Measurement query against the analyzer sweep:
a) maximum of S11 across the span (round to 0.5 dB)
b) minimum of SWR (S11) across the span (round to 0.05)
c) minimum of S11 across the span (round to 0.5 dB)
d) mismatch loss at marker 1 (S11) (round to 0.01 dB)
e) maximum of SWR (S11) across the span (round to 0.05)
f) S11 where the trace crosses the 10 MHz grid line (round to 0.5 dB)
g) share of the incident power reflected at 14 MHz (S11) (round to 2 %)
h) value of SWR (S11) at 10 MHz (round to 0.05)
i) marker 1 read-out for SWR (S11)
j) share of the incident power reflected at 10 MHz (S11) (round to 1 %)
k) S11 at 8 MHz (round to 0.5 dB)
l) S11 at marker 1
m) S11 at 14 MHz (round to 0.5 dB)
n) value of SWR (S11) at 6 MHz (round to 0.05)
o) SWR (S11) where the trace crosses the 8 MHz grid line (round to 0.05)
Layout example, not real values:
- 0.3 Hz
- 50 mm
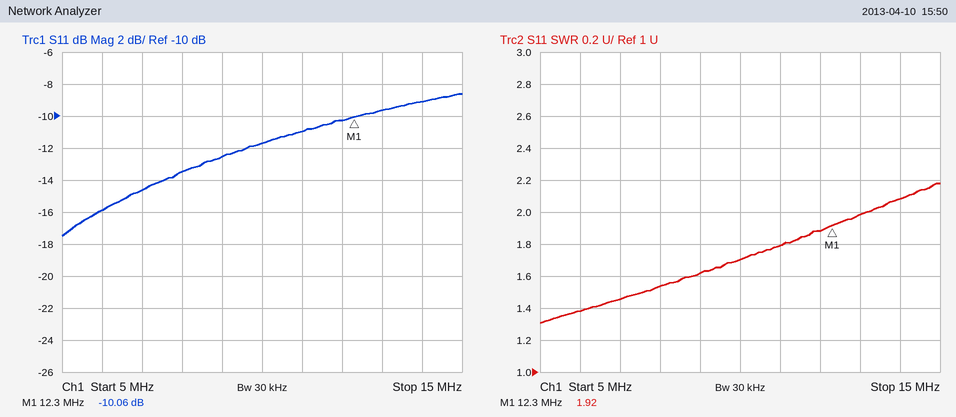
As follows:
- -8.5 dB
- 1.30
- -17.5 dB
- 0.45 dB
- 2.20
- -11.5 dB
- 12 %
- 1.70
- 1.92
- 7 %
- -13.5 dB
- -10.06 dB
- -9.0 dB
- 1.40
- 1.55
